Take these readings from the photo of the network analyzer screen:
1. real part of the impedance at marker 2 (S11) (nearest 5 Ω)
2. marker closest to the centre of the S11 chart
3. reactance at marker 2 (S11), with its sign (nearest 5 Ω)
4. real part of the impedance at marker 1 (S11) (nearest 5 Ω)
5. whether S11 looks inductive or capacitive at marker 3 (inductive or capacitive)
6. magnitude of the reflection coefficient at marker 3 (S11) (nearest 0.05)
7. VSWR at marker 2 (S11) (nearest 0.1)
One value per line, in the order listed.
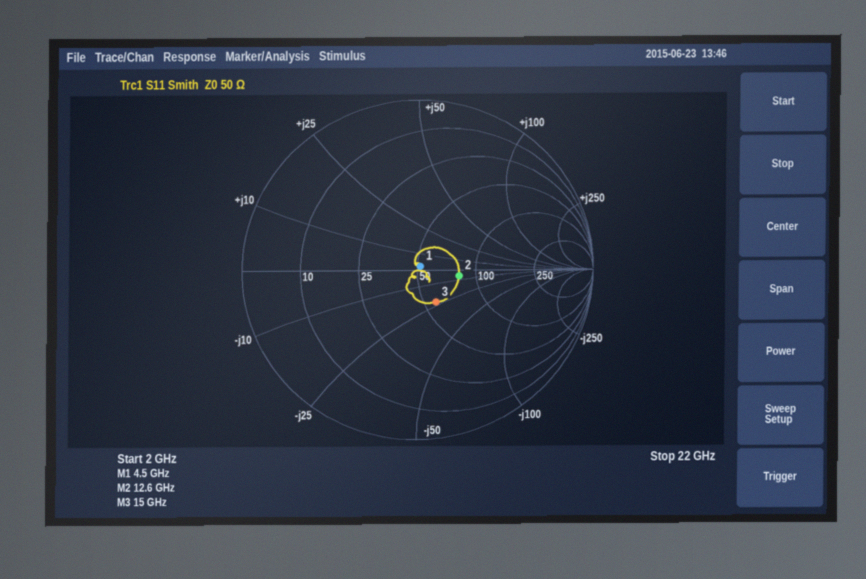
80 Ω
marker 1
-5 Ω
50 Ω
capacitive
0.20
1.6
